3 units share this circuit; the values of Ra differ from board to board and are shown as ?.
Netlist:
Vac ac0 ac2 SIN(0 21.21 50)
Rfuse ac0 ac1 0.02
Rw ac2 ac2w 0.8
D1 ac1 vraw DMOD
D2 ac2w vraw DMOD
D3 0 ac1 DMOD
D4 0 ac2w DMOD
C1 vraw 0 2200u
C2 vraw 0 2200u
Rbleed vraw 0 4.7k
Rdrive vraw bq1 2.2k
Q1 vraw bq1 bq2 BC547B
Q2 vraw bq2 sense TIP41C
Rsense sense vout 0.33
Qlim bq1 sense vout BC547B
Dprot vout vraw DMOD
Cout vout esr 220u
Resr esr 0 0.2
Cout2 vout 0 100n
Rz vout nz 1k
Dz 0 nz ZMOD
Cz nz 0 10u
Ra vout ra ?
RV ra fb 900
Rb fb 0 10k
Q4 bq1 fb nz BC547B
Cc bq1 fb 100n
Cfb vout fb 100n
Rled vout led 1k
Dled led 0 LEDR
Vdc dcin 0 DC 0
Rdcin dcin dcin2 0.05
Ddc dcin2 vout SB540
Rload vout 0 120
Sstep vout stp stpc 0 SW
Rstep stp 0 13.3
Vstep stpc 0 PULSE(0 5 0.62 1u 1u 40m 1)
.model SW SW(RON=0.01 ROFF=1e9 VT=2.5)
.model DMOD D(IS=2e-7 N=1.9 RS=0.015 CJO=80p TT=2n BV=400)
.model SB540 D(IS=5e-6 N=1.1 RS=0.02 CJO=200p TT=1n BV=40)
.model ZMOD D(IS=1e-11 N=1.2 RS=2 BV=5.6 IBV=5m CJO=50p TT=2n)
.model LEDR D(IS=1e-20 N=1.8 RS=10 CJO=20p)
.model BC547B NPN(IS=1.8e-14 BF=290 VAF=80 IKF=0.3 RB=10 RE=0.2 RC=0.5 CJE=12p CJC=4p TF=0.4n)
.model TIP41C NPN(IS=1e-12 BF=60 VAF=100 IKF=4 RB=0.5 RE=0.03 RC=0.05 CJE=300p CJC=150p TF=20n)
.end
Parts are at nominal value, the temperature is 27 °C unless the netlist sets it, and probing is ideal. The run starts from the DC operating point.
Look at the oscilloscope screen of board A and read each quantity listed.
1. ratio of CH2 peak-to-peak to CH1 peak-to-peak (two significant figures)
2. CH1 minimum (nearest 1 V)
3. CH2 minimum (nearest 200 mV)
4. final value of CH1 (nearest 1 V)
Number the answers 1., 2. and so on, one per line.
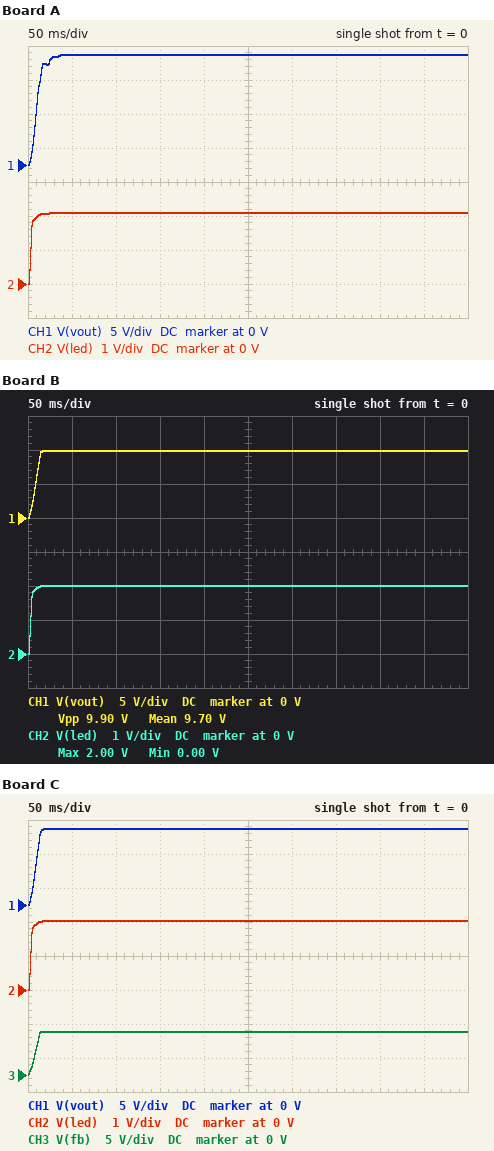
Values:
1. 0.13
2. 0 V
3. 0 V
4. 16 V
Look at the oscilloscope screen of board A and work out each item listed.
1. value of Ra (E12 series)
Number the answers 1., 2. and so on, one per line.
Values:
1. 15 kΩ
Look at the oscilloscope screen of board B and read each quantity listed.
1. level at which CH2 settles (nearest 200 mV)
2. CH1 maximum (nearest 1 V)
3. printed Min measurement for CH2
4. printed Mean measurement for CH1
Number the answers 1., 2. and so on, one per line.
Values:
1. 2.0 V
2. 10 V
3. 0.00 V
4. 9.70 V
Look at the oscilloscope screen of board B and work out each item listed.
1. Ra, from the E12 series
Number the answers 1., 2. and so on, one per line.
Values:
1. 4.7 kΩ
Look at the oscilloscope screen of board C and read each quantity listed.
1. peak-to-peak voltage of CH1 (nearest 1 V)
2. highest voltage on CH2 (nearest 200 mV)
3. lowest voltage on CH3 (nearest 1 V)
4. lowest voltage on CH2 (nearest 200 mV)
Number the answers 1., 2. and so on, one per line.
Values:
1. 11 V
2. 2.0 V
3. 0 V
4. 0 V
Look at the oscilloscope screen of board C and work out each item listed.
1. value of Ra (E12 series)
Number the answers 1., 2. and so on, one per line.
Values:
1. 6.8 kΩ
